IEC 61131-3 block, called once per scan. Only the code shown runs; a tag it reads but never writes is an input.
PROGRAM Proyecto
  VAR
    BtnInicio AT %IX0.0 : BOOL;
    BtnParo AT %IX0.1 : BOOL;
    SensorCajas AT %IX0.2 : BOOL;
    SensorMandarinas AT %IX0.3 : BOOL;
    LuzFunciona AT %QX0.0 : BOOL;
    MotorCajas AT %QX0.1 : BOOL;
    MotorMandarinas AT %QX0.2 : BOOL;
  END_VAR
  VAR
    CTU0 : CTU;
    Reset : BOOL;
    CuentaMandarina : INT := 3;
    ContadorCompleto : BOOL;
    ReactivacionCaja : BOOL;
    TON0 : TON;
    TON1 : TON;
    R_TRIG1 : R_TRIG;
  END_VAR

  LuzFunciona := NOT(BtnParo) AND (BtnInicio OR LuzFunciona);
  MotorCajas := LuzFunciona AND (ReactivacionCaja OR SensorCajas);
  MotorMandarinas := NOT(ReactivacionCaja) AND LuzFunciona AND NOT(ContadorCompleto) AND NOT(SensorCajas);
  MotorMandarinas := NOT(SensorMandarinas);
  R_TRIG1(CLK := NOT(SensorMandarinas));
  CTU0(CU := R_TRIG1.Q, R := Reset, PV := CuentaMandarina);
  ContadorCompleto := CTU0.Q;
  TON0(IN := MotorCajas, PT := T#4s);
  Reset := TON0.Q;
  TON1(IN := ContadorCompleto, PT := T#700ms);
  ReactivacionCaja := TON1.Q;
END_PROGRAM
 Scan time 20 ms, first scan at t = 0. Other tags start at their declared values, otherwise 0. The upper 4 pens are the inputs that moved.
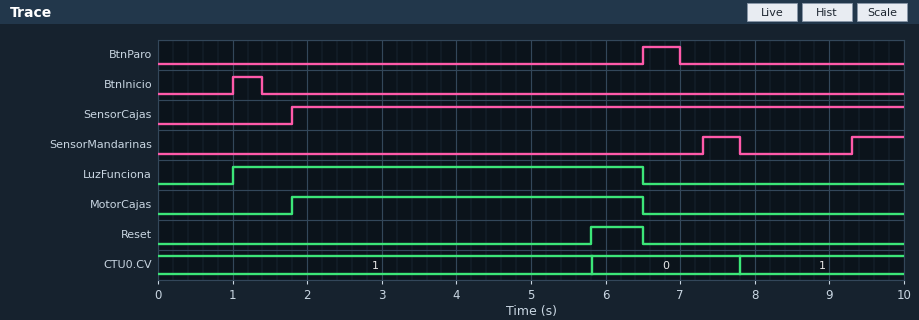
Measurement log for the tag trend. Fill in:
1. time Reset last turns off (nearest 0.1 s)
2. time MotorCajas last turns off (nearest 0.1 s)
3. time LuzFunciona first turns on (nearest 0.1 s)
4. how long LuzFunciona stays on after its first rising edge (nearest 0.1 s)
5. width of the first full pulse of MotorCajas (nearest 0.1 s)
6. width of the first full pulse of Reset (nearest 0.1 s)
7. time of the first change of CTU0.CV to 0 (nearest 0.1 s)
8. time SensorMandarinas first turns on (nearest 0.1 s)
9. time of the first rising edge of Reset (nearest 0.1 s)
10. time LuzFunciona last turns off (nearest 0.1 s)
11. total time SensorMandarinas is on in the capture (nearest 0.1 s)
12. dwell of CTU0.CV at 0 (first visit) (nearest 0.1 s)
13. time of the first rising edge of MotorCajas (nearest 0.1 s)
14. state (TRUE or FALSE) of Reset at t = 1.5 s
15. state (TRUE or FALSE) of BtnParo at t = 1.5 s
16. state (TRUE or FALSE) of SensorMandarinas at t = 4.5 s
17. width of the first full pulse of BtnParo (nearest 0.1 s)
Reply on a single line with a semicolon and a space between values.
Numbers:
6.5 s; 6.5 s; 1.0 s; 5.5 s; 4.7 s; 0.7 s; 5.8 s; 7.3 s; 5.8 s; 6.5 s; 1.2 s; 2.0 s; 1.8 s; FALSE; FALSE; FALSE; 0.5 s
